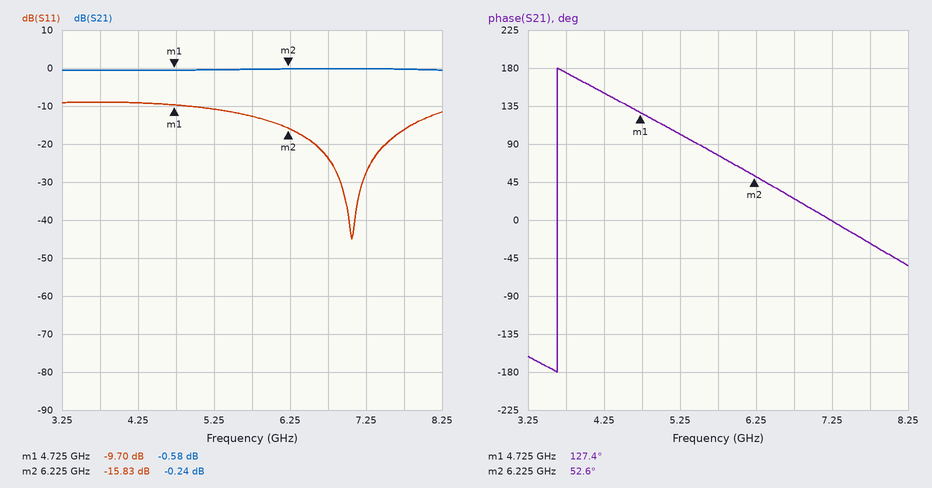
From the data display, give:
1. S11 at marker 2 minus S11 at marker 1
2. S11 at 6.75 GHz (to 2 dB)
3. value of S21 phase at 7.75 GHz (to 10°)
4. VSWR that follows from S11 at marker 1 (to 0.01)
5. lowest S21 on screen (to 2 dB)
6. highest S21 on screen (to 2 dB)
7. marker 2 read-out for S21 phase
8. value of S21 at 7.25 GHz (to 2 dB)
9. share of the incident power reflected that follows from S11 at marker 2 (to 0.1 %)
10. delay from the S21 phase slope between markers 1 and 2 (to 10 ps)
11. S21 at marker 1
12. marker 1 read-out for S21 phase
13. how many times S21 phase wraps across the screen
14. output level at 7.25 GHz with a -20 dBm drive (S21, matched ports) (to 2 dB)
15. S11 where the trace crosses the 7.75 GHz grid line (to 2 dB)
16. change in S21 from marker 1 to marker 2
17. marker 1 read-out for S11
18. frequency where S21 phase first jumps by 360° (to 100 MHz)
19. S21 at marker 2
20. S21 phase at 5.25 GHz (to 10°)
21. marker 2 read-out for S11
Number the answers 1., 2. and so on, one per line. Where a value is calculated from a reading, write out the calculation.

1. -15.83 − (-9.7) = -6.13 dB
2. -24 dB
3. -30°
4. (1 + 0.3273)/(1 − 0.3273) ≈ 1.97
5. 0 dB
6. 0 dB
7. 52.6°
8. 0 dB
9. 10^(-15.83/10) ≈ 2.6 %
10. −(52.6° − (127.4°))/(360° × 1.5 GHz) ≈ 139 ps, so 140 ps to the nearest 10 ps
11. -0.58 dB
12. 127.4°
13. 1
14. -20 dBm + (0 dB) = -20 dBm
15. -16 dB
16. -0.24 − (-0.58) = 0.34 dB
17. -9.70 dB
18. 3.6 GHz
19. -0.24 dB
20. 100°
21. -15.83 dB
